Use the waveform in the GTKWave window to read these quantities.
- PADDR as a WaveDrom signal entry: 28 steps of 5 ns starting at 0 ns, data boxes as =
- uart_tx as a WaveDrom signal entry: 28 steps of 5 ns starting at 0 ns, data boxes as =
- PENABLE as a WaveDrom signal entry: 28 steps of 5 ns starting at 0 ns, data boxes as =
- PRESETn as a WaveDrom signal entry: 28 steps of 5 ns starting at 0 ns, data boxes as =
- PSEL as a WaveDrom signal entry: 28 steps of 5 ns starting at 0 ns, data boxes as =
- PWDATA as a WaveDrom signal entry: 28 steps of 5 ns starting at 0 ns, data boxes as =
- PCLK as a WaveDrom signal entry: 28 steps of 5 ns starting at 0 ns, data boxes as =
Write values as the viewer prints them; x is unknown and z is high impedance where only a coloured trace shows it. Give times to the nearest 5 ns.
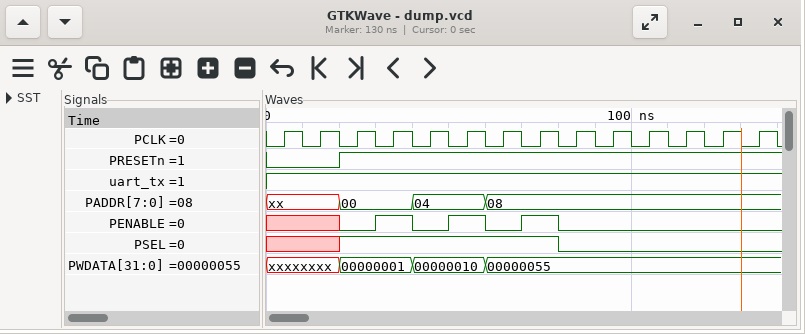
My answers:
{name: 'PADDR', wave: 'x...=...=...=...............', data: '00 04 08'}
{name: 'uart_tx', wave: '1...........................'}
{name: 'PENABLE', wave: 'x...0.1.0.1.0.1.0...........'}
{name: 'PRESETn', wave: '0...1.......................'}
{name: 'PSEL', wave: 'x...1...........0...........'}
{name: 'PWDATA', wave: 'x...=...=...=...............', data: '00000001 00000010 00000055'}
{name: 'PCLK', wave: '0101010101010101010101010101'}
